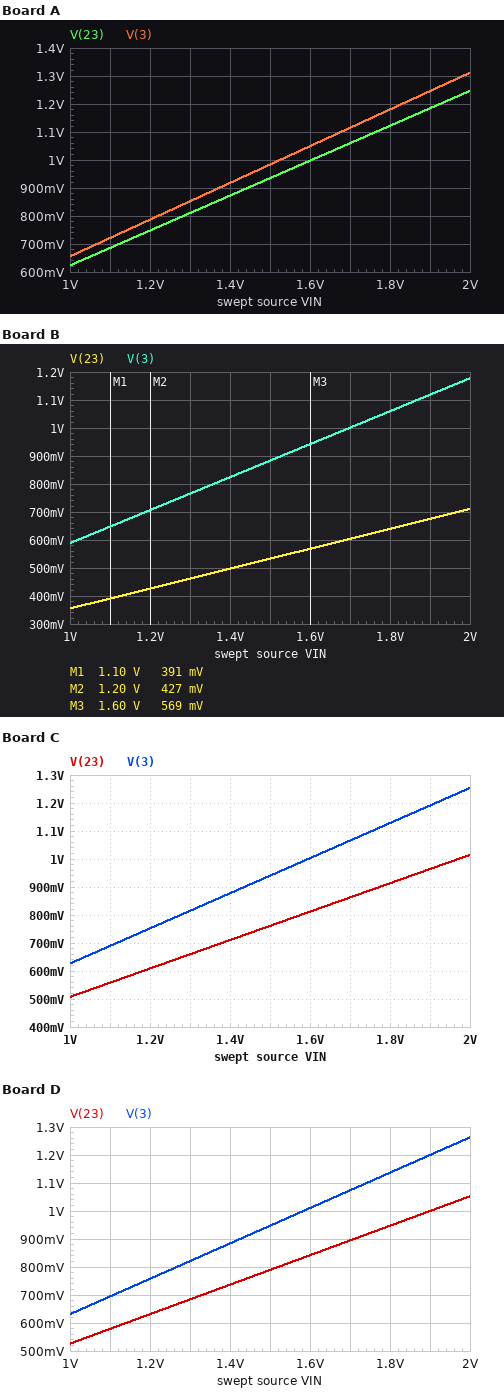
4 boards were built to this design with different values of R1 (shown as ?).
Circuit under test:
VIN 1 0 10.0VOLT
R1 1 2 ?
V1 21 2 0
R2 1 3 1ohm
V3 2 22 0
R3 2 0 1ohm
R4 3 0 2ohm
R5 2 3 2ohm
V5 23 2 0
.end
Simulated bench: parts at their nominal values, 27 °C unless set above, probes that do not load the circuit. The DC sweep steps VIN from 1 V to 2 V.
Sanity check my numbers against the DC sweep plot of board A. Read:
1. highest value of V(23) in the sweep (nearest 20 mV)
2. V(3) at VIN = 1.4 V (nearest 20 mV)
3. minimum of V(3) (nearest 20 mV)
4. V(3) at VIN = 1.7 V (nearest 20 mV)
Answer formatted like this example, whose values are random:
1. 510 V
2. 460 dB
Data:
1. 1.24 V
2. 920 mV
3. 660 mV
4. 1.12 V
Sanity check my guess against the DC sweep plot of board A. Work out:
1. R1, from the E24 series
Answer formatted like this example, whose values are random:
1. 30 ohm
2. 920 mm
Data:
1. 0.62 Ω
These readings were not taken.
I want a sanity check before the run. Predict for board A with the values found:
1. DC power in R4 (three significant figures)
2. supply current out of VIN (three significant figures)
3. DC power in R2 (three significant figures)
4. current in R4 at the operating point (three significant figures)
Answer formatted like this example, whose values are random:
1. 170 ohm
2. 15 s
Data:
1. 21.5 W
2. 9.51 A
3. 11.8 W
4. 3.28 A
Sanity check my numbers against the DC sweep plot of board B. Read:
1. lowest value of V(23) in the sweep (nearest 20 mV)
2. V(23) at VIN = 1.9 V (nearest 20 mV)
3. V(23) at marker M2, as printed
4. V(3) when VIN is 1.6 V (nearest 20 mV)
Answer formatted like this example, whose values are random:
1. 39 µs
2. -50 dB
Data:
1. 360 mV
2. 680 mV
3. 427 mV
4. 940 mV
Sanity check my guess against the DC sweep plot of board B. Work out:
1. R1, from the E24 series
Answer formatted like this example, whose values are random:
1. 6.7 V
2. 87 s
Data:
1. 2.7 Ω
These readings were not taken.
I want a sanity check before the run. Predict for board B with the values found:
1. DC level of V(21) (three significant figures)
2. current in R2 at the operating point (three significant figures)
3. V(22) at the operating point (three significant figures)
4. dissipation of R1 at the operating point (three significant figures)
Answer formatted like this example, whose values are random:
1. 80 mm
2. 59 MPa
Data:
1. 3.55 V
2. 4.11 A
3. 3.55 V
4. 15.4 W
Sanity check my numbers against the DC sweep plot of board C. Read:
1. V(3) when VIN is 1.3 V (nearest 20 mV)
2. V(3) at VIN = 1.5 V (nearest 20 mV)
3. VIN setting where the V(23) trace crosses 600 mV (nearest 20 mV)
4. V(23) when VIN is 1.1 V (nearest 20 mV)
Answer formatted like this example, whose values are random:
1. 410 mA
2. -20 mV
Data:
1. 820 mV
2. 940 mV
3. 1.18 V
4. 560 mV
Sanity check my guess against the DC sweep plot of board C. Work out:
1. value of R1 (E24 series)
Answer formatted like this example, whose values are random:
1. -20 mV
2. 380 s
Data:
1. 1.1 Ω
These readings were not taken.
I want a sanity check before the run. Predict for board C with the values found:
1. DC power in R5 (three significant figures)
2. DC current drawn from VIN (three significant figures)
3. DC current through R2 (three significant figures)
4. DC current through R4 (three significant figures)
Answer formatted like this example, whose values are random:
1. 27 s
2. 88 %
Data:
1. 713 mW
2. 8.21 A
3. 3.73 A
4. 3.13 A
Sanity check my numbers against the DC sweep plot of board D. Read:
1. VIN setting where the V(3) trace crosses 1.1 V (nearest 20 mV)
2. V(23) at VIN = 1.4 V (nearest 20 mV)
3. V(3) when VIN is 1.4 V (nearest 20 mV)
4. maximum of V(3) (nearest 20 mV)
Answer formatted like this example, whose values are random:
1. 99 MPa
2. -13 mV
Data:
1. 1.74 V
2. 740 mV
3. 880 mV
4. 1.26 V
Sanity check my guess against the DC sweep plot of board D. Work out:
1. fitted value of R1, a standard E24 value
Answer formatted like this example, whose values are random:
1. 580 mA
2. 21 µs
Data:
1. 1 Ω
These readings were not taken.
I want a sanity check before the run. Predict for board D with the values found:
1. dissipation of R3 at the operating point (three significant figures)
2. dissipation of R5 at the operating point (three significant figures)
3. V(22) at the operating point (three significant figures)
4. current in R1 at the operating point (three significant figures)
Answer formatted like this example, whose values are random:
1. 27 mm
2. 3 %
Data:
1. 27.7 W
2. 554 mW
3. 5.26 V
4. 4.74 A
